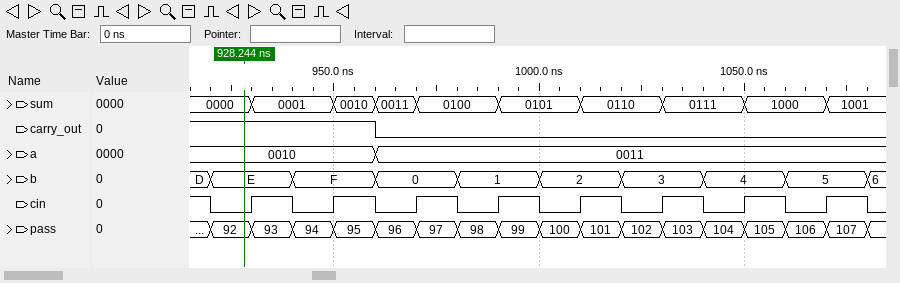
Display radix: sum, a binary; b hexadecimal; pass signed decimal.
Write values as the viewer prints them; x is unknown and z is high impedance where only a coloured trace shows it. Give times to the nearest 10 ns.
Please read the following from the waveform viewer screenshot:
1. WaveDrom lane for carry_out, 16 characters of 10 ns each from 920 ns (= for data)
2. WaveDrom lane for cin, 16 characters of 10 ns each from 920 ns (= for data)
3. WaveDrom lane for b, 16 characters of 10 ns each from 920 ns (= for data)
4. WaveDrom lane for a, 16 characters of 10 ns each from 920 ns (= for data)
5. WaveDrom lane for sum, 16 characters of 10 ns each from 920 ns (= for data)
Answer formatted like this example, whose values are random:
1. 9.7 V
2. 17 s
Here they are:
1. {name: 'carry_out', wave: '1...0...........'}
2. {name: 'cin', wave: '0101010101010101'}
3. {name: 'b', wave: '=.=.=.=.=.=.=.=.', data: 'E F 0 1 2 3 4 5'}
4. {name: 'a', wave: '=...=...........', data: '0010 0011'}
5. {name: 'sum', wave: '==.===.=.=.=.=.=', data: '0000 0001 0010 0011 0100 0101 0110 0111 1000 1001'}
